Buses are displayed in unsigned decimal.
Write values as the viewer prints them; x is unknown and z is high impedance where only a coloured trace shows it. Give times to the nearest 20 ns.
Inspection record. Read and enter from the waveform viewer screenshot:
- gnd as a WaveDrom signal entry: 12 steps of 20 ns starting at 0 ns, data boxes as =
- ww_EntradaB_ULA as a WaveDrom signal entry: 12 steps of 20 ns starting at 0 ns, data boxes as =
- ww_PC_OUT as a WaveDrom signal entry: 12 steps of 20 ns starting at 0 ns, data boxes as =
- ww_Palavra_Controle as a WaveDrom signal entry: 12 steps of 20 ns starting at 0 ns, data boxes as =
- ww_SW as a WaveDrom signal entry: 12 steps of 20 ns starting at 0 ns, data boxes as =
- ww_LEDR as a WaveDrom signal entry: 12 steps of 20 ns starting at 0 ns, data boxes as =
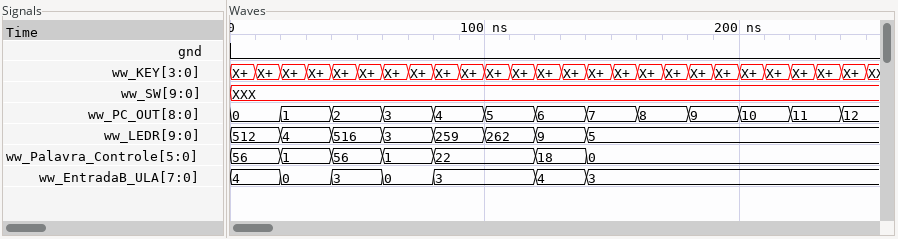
{name: 'gnd', wave: '0...........'}
{name: 'ww_EntradaB_ULA', wave: '=====.==....', data: '4 0 3 0 3 4 3'}
{name: 'ww_PC_OUT', wave: '============', data: '0 1 2 3 4 5 6 7 8 9 10 11'}
{name: 'ww_Palavra_Controle', wave: '=====.==....', data: '56 1 56 1 22 18 0'}
{name: 'ww_SW', wave: 'x...........'}
{name: 'ww_LEDR', wave: '========....', data: '512 4 516 3 259 262 9 5'}
